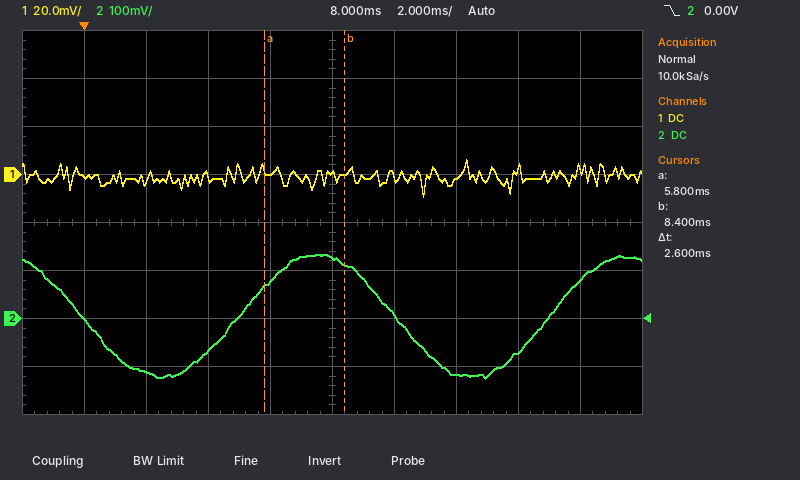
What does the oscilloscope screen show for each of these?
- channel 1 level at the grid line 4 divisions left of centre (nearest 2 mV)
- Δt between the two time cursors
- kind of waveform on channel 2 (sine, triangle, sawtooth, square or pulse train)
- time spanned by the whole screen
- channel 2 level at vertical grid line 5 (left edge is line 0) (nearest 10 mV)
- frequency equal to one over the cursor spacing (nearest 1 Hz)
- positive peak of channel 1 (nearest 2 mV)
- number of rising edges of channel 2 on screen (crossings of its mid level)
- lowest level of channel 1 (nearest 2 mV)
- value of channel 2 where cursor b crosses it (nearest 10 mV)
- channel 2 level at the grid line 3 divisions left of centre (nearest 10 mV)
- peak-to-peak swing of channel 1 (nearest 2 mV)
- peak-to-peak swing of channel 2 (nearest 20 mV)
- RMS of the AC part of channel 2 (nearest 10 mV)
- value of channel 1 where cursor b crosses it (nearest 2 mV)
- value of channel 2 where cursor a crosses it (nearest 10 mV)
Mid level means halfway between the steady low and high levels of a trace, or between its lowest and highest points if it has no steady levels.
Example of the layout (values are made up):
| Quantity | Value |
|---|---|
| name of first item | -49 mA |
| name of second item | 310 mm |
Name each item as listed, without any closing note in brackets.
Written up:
| Quantity | Value |
|---|---|
| channel 1 level at the grid line 4 divisions left of centre | 0 mV |
| Δt between the two time cursors | 2.6 ms |
| kind of waveform on channel 2 | sine |
| time spanned by the whole screen | 20 ms |
| channel 2 level at vertical grid line 5 (left edge is line 0) | 130 mV |
| frequency equal to one over the cursor spacing | 385 Hz |
| positive peak of channel 1 | 6 mV |
| number of rising edges of channel 2 on screen | 2 |
| lowest level of channel 1 | -10 mV |
| value of channel 2 where cursor b crosses it | 110 mV |
| channel 2 level at the grid line 3 divisions left of centre | -110 mV |
| peak-to-peak swing of channel 1 | 16 mV |
| peak-to-peak swing of channel 2 | 260 mV |
| RMS of the AC part of channel 2 | 90 mV |
| value of channel 1 where cursor b crosses it | 0 mV |
| value of channel 2 where cursor a crosses it | 70 mV |
